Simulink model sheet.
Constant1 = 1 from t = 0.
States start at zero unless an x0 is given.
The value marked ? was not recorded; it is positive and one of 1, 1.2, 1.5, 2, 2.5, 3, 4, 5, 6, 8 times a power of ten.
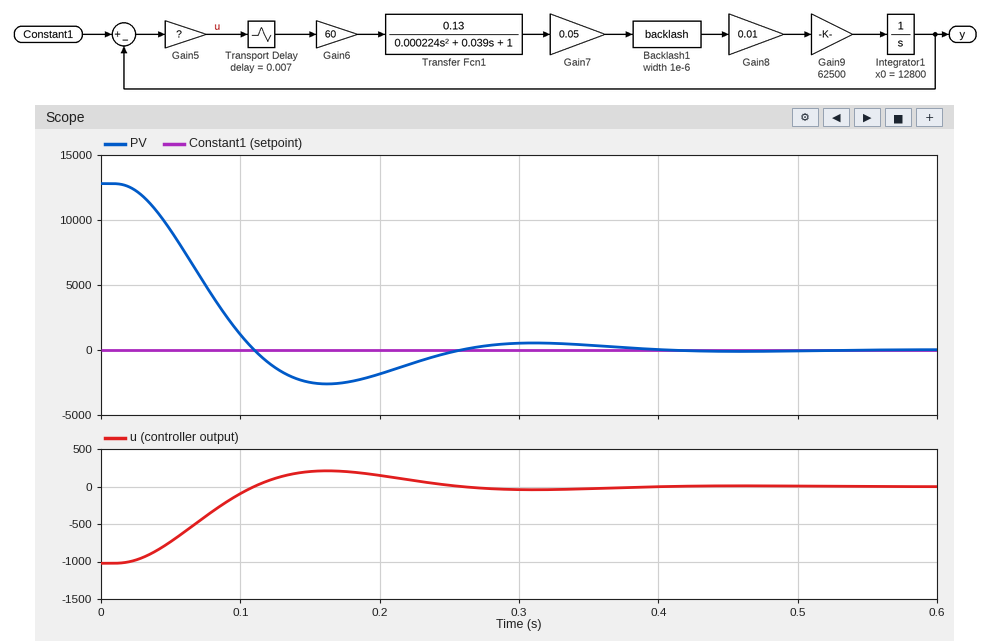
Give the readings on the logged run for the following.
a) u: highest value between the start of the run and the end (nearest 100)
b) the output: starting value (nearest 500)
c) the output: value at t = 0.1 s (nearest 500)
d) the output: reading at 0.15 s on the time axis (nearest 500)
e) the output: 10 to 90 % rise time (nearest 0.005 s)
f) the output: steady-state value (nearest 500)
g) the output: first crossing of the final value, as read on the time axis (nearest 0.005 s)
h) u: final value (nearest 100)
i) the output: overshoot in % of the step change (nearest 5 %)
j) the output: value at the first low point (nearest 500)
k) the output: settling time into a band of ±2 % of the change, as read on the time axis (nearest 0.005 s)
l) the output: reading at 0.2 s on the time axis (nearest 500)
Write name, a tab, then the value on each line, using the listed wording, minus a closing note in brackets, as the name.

u: highest value between the start of the run and the end	200
the output: starting value	13000
the output: value at t = 0.1 s	1000
the output: reading at 0.15 s on the time axis	-2500
the output: 10 to 90 % rise time	0.065 s
the output: steady-state value	0
the output: first crossing of the final value, as read on the time axis	0.110 s
u: final value	0
the output: overshoot in % of the step change	20 %
the output: value at the first low point	-2500
the output: settling time into a band of ±2 % of the change, as read on the time axis	0.365 s
the output: reading at 0.2 s on the time axis	-2000
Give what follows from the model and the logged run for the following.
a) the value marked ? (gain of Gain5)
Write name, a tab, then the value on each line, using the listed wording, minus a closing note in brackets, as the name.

the value marked ?	0.08
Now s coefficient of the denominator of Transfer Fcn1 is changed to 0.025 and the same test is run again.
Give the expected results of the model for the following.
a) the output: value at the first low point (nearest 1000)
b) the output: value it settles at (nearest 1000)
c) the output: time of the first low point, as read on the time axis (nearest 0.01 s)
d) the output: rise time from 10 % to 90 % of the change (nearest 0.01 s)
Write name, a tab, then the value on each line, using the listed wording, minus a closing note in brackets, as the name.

the output: value at the first low point	-2000
the output: value it settles at	0
the output: time of the first low point, as read on the time axis	0.13 s
the output: rise time from 10 % to 90 % of the change	0.06 s
